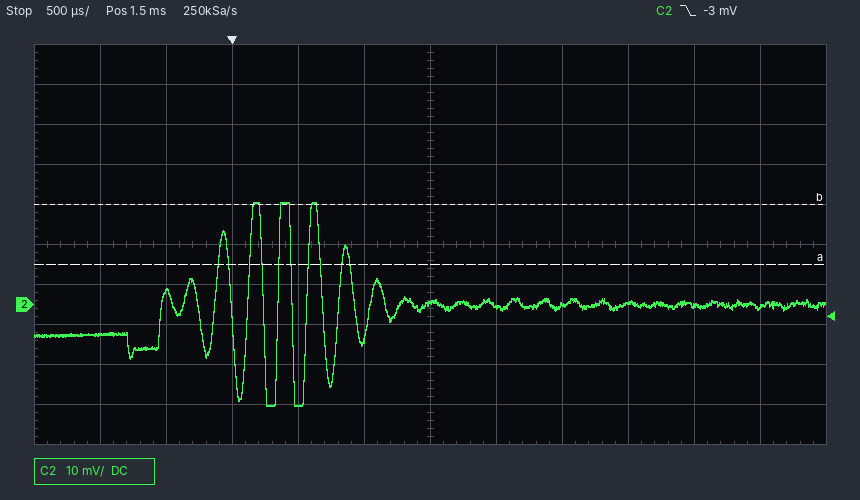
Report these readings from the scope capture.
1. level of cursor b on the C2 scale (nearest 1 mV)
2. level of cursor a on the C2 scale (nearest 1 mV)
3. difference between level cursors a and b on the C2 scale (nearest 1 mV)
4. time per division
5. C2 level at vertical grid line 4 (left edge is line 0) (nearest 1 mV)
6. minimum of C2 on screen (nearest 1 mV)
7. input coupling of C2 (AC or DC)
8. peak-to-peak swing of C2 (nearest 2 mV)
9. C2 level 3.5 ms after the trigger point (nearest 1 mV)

25 mV
10 mV
15 mV
500 µs
-25 mV
-25 mV
DC
50 mV
0 mV
